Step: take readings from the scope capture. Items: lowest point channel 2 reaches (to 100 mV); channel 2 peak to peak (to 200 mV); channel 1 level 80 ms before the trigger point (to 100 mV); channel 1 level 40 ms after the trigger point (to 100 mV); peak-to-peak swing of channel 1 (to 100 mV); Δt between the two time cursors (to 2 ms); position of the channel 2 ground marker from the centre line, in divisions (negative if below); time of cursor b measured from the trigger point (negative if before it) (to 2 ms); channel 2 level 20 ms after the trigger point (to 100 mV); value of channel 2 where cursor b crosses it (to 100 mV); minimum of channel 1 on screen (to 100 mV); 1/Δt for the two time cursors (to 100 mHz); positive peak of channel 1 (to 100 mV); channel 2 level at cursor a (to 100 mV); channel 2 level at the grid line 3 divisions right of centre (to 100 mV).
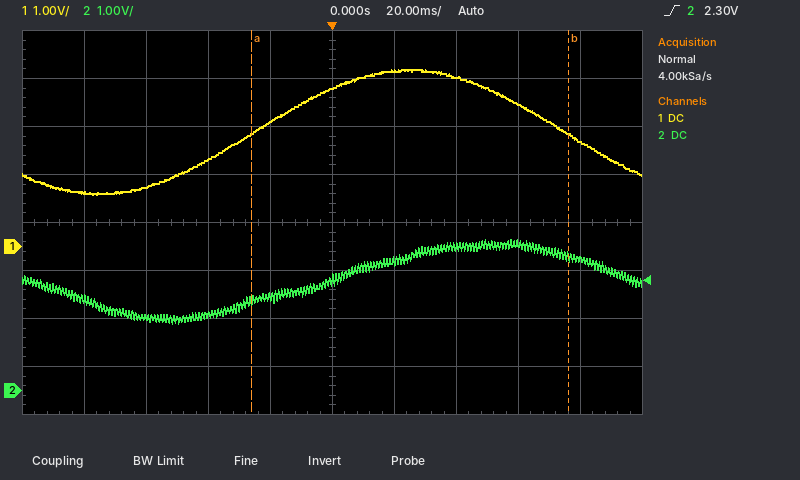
1.4 V
1.8 V
1.1 V
3.5 V
2.6 V
102 ms
-3.5 div
+76 ms
2.7 V
2.8 V
1.1 V
9.8 Hz
3.7 V
1.9 V
3.1 V
